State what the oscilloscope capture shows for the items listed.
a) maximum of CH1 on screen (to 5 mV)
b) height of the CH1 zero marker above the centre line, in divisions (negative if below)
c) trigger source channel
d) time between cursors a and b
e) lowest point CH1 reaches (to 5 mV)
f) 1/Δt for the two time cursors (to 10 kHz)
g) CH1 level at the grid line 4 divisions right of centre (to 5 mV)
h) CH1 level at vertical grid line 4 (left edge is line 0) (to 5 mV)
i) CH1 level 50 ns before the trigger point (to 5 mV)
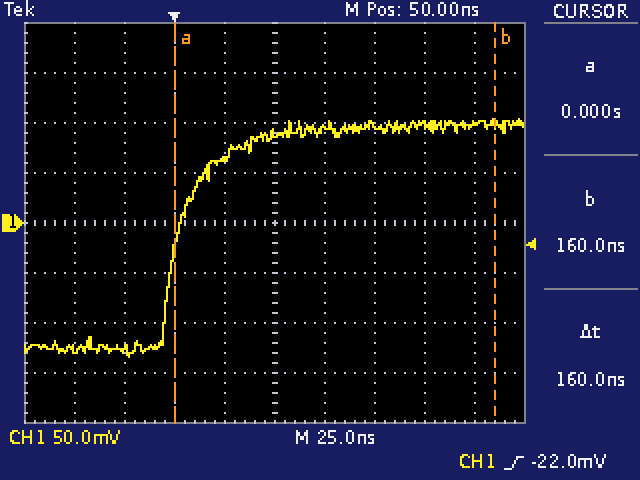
105 mV
0.0 div
CH1
160 ns
-135 mV
6.25 MHz
100 mV
65 mV
-125 mV
